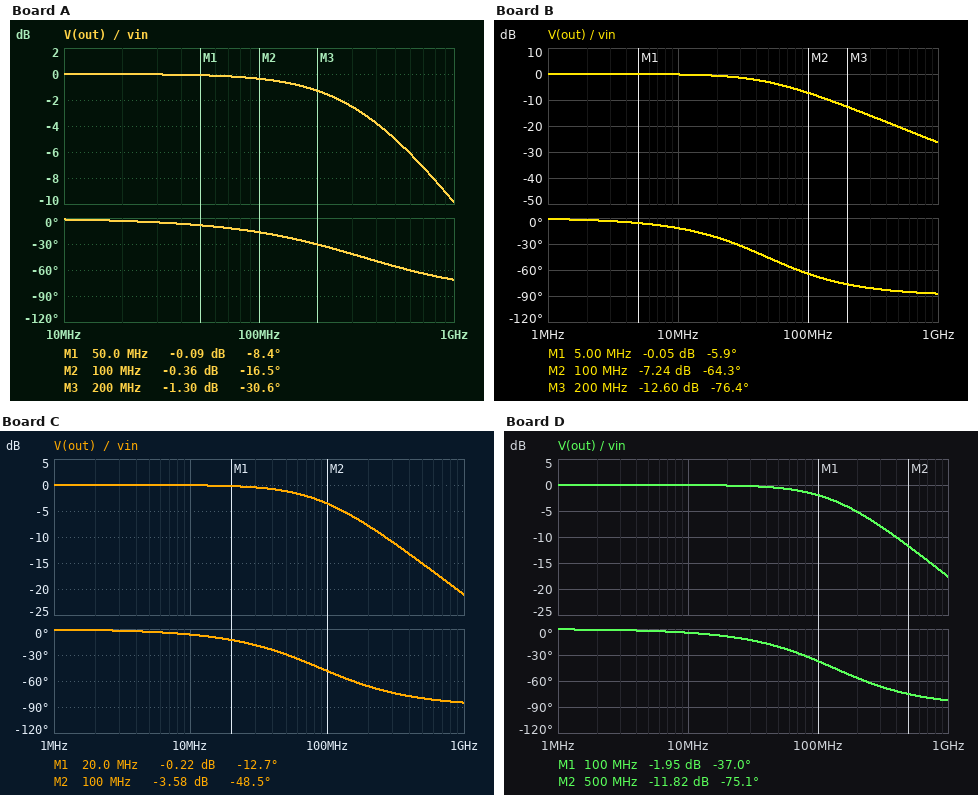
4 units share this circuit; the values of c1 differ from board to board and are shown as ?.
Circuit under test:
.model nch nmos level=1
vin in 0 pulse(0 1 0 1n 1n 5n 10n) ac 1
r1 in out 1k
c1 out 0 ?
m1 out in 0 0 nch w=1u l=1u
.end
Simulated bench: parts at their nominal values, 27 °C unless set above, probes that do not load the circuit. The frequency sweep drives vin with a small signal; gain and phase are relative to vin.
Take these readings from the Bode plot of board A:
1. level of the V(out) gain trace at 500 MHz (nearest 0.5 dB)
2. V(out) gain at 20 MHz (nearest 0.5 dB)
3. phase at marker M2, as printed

-5.0 dB
0 dB
-16.5 deg
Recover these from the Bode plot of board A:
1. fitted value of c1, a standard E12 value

470 fF
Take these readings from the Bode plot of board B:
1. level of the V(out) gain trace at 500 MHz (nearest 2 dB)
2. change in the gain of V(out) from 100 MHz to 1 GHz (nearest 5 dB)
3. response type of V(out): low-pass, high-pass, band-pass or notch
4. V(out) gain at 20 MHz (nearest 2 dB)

-20 dB
-20 dB
low-pass
0 dB
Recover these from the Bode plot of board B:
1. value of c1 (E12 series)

3.3 pF
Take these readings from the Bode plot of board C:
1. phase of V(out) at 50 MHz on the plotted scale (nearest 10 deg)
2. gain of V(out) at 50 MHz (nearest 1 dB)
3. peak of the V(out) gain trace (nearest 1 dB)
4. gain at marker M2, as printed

-30 deg
-1 dB
0 dB
-3.58 dB
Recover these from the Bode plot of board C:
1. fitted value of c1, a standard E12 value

1.8 pF
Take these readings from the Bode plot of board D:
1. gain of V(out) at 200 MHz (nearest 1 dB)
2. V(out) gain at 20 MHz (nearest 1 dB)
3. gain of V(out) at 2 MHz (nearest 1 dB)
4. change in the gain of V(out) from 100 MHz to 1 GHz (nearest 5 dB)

-5 dB
0 dB
0 dB
-15 dB
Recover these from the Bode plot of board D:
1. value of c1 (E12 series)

1.2 pF
